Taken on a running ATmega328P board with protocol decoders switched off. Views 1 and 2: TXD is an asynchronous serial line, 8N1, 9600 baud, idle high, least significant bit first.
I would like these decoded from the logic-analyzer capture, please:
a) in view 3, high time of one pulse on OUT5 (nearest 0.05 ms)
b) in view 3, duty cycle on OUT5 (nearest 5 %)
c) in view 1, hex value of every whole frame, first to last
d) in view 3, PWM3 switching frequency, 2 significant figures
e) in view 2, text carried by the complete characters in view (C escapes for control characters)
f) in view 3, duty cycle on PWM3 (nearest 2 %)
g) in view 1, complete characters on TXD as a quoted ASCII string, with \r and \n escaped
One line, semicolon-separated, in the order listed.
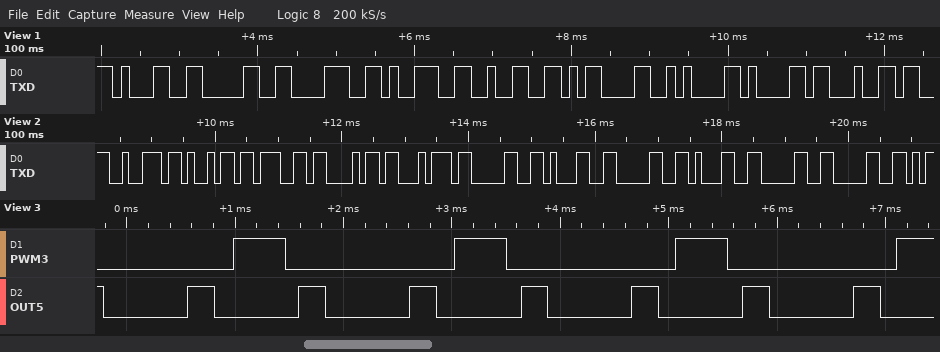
0.25 ms; 25 %; 0x31 0x30 0x38 0x39 0x32 0x0D 0x0A 0x61 0x64; 490 Hz; "right010100"; 24 %; "10892\r\nad"
